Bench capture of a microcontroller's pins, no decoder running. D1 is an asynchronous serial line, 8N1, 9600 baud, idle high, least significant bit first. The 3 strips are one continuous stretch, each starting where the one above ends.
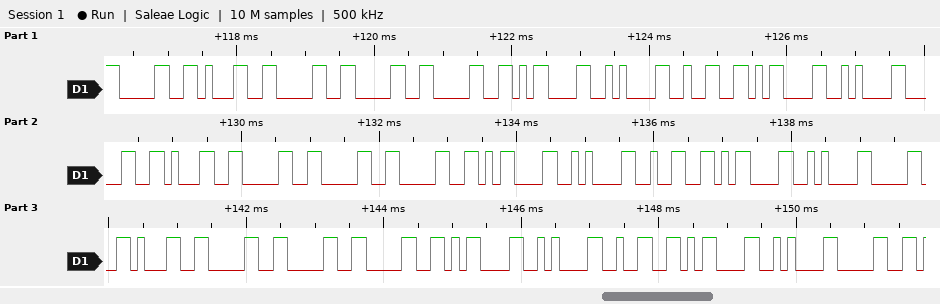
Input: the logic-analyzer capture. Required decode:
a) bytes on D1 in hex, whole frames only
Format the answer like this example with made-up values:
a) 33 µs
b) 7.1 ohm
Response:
a) 30 31 30 30 30 0D 0A 32 0D 0A 30 31 30 30 30 0D 0A 32 0D 0A 30 31 30 30 30 0D 0A 32 0D 0A 30
